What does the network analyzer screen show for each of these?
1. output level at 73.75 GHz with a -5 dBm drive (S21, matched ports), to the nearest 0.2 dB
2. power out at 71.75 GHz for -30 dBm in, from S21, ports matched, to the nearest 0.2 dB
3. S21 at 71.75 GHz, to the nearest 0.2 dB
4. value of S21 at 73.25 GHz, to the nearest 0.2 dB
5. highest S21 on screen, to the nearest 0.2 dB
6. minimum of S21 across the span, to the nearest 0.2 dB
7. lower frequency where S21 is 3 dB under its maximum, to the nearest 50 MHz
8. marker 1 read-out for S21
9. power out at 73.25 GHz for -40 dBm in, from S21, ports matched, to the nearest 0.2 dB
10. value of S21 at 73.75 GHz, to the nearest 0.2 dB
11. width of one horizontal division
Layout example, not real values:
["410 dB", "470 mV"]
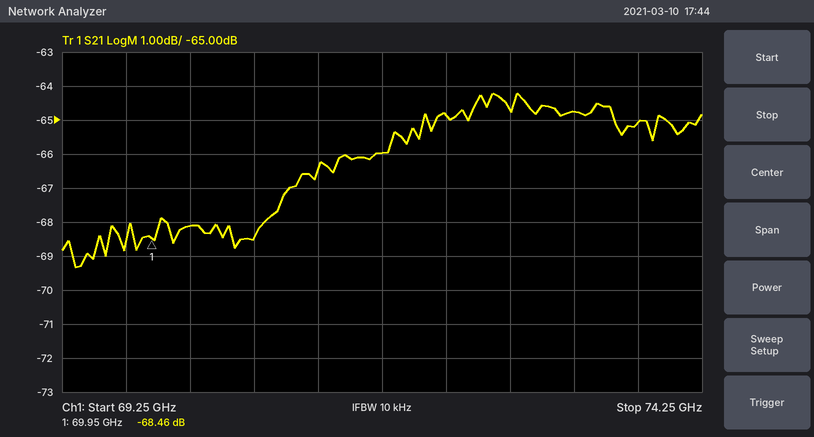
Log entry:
["-70.0 dBm", "-96.0 dBm", "-66.0 dB", "-64.8 dB", "-64.2 dB", "-69.4 dB", "71.00 GHz", "-68.46 dB", "-104.8 dBm", "-65.0 dB", "500 MHz"]
